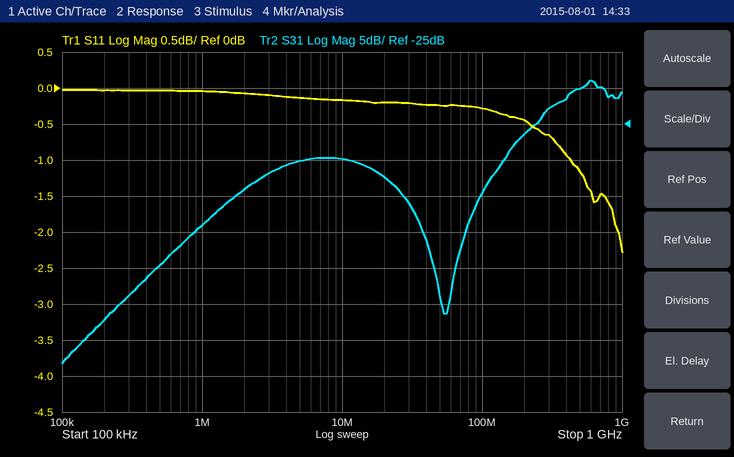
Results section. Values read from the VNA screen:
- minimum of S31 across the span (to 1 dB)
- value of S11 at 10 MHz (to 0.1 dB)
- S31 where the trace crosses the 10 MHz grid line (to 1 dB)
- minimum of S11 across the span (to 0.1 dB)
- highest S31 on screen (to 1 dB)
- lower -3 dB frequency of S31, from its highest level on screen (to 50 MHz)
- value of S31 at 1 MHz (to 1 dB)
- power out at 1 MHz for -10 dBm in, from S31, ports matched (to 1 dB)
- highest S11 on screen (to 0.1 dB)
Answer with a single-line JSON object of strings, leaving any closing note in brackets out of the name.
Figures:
{"minimum of S31 across the span": "-58 dB", "value of S11 at 10 MHz": "-0.2 dB", "S31 where the trace crosses the 10 MHz grid line": "-30 dB", "minimum of S11 across the span": "-2.3 dB", "highest S31 on screen": "-19 dB", "lower -3 dB frequency of S31, from its highest level on screen": "350 MHz", "value of S31 at 1 MHz": "-39 dB", "power out at 1 MHz for -10 dBm in, from S31, ports matched": "-49 dBm", "highest S11 on screen": "0.0 dB"}
